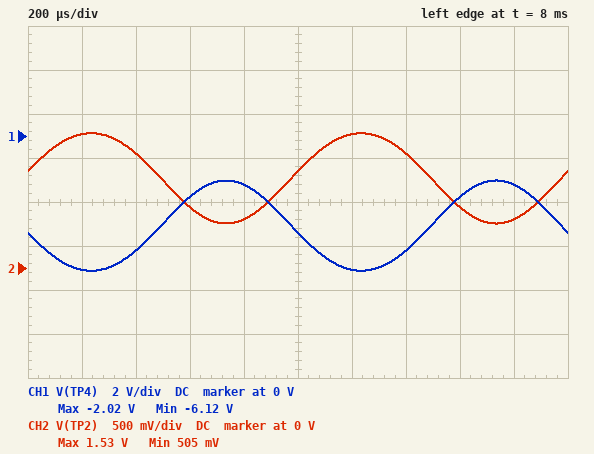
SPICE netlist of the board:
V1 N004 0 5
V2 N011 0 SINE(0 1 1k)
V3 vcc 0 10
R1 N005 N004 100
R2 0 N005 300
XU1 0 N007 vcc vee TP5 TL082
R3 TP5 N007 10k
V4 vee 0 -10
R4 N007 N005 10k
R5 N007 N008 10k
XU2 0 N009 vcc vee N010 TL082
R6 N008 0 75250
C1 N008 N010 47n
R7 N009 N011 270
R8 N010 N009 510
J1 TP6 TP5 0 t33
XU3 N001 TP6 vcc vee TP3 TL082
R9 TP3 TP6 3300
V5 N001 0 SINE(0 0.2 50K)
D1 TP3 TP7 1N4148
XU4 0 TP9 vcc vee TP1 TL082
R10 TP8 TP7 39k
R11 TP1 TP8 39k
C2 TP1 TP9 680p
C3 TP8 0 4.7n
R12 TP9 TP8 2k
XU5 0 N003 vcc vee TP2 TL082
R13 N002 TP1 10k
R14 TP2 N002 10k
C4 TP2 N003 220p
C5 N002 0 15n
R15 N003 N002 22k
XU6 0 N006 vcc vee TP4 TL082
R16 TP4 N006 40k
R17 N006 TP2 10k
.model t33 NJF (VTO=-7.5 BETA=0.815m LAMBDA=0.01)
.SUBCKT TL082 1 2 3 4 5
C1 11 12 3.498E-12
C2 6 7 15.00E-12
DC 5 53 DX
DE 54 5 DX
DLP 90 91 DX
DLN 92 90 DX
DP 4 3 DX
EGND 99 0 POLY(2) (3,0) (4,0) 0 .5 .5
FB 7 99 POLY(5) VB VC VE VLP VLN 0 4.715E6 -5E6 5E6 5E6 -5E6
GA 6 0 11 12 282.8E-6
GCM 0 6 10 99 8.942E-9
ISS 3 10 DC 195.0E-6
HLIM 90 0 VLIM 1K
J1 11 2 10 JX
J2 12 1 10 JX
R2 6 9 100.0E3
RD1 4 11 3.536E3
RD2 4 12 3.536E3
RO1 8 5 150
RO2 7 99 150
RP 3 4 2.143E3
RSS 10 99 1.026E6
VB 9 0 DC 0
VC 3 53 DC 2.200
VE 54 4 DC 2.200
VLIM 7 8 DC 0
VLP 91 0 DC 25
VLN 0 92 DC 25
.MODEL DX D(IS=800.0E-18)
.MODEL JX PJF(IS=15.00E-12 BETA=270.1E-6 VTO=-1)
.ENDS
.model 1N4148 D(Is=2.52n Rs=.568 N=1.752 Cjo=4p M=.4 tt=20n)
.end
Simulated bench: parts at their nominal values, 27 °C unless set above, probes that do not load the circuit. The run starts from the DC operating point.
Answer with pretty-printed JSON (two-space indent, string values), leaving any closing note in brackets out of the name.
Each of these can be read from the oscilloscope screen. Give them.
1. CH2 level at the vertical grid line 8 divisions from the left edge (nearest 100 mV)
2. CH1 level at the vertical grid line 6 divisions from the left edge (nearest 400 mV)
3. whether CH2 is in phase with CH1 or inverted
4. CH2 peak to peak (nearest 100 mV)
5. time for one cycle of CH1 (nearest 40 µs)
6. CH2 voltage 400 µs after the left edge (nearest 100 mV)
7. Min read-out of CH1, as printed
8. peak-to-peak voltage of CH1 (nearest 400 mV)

{
  "CH2 level at the vertical grid line 8 divisions from the left edge": "700 mV",
  "CH1 level at the vertical grid line 6 divisions from the left edge": "-6.0 V",
  "whether CH2 is in phase with CH1 or inverted": "inverted",
  "CH2 peak to peak": "1.0 V",
  "time for one cycle of CH1": "1.00 ms",
  "CH2 voltage 400 µs after the left edge": "1.3 V",
  "Min read-out of CH1, as printed": "-6.12 V",
  "peak-to-peak voltage of CH1": "4.0 V"
}
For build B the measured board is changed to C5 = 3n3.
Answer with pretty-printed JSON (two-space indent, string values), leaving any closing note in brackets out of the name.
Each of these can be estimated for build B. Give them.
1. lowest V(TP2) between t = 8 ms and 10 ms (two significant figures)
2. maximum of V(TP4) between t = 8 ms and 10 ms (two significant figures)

{
  "lowest V(TP2) between t = 8 ms and 10 ms": "520 mV",
  "maximum of V(TP4) between t = 8 ms and 10 ms": "-2.1 V"
}
